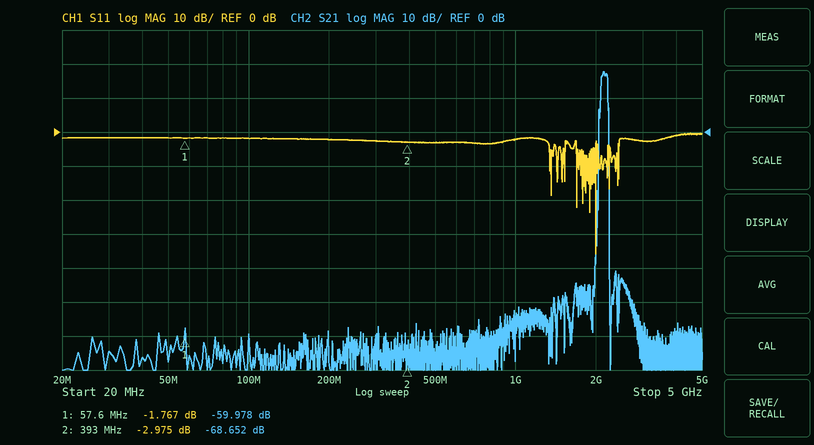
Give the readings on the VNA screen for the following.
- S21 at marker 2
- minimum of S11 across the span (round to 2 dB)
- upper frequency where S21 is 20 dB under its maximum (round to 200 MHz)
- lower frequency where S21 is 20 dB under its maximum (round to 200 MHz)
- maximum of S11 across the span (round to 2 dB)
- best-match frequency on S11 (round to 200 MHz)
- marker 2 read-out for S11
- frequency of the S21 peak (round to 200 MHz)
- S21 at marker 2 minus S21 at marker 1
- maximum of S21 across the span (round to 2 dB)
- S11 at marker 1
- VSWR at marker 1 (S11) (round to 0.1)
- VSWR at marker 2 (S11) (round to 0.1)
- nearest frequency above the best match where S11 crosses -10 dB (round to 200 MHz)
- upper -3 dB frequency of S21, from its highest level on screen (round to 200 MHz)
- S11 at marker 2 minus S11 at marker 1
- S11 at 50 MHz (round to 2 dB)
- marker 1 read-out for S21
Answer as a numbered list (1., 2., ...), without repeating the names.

1. -68.652 dB
2. -36 dB
3. 2.2 GHz
4. 2.0 GHz
5. 0 dB
6. 2.0 GHz
7. -2.975 dB
8. 2.2 GHz
9. -8.674 dB
10. 18 dB
11. -1.767 dB
12. 9.9
13. 5.9
14. 2.0 GHz
15. 2.2 GHz
16. -1.208 dB
17. -2 dB
18. -59.978 dB
